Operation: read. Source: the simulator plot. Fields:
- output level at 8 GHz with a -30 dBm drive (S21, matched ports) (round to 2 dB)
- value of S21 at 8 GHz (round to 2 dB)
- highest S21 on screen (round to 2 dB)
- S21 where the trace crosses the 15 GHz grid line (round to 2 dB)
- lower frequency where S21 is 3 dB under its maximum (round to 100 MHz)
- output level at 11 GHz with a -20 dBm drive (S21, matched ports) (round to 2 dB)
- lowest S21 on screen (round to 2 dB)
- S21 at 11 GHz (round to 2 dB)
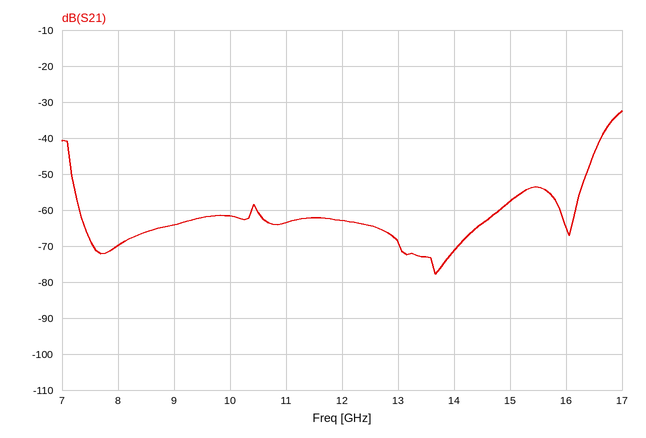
-100 dBm
-70 dB
-32 dB
-58 dB
16.8 GHz
-84 dBm
-78 dB
-64 dB
